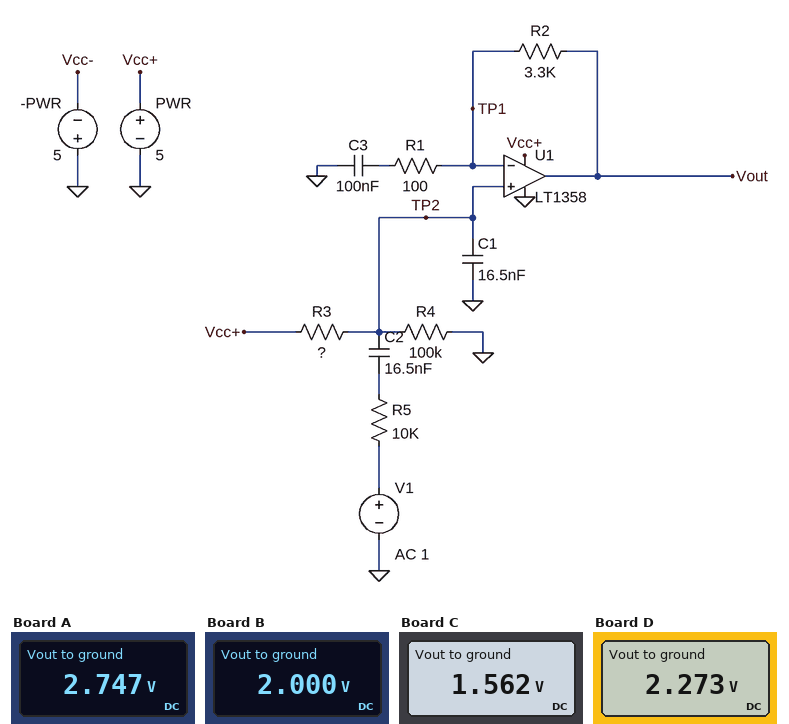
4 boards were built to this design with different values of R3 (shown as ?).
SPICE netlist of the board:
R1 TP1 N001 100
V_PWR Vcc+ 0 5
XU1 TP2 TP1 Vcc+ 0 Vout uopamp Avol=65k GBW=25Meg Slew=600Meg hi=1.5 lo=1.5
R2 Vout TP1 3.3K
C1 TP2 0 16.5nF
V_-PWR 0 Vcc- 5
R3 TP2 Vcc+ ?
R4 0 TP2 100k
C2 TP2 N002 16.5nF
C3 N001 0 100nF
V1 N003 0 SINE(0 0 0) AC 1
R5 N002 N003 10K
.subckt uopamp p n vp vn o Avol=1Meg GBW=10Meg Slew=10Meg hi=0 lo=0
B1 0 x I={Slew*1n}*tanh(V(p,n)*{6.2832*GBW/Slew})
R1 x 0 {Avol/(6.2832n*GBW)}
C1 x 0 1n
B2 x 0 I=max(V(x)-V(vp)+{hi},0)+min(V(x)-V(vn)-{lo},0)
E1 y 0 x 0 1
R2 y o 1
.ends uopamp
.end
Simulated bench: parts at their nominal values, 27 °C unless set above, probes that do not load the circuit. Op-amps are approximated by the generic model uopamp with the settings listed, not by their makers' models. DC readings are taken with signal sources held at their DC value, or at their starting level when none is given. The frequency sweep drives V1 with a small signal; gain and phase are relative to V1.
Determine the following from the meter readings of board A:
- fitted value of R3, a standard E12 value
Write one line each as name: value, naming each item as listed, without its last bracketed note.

fitted value of R3, a standard E12 value: 82 kΩ
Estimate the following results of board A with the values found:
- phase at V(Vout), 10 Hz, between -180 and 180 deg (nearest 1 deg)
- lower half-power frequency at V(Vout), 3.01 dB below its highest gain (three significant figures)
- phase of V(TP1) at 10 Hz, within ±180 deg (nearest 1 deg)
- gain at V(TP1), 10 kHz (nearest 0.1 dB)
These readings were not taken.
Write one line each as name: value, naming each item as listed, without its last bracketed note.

phase at V(Vout), 10 Hz, between -180 and 180 deg: 85 deg
lower half-power frequency at V(Vout), 3.01 dB below its highest gain: 1.56 kHz
phase of V(TP1) at 10 Hz, within ±180 deg: 84 deg
gain at V(TP1), 10 kHz: -20.4 dB
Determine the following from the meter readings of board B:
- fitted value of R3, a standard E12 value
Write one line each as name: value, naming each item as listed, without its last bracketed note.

fitted value of R3, a standard E12 value: 150 kΩ
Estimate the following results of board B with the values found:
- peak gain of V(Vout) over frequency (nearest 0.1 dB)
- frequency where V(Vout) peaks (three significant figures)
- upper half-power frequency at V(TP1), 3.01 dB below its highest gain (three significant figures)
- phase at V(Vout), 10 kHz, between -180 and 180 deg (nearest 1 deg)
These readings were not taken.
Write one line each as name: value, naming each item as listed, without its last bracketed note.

peak gain of V(Vout) over frequency: 5.3 dB
frequency where V(Vout) peaks: 5.62 kHz
upper half-power frequency at V(TP1), 3.01 dB below its highest gain: 2.16 kHz
phase at V(Vout), 10 kHz, between -180 and 180 deg: -23 deg
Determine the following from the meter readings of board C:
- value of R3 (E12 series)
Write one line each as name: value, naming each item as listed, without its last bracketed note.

value of R3: 220 kΩ
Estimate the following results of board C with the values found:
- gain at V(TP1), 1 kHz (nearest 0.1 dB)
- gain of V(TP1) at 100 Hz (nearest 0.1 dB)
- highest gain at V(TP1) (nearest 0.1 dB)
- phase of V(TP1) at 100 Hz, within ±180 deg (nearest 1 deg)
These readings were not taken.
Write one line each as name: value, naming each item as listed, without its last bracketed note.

gain at V(TP1), 1 kHz: -7.3 dB
gain of V(TP1) at 100 Hz: -8.0 dB
highest gain at V(TP1): -6.6 dB
phase of V(TP1) at 100 Hz, within ±180 deg: 31 deg
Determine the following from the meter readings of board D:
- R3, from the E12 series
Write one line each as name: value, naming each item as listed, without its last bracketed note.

R3, from the E12 series: 120 kΩ
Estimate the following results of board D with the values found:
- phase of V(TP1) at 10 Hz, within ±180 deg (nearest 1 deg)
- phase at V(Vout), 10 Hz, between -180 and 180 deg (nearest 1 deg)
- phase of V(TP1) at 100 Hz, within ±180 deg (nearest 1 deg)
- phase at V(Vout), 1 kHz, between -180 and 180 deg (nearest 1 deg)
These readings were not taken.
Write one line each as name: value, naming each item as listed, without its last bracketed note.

phase of V(TP1) at 10 Hz, within ±180 deg: 83 deg
phase at V(Vout), 10 Hz, between -180 and 180 deg: 84 deg
phase of V(TP1) at 100 Hz, within ±180 deg: 37 deg
phase at V(Vout), 1 kHz, between -180 and 180 deg: 40 deg
